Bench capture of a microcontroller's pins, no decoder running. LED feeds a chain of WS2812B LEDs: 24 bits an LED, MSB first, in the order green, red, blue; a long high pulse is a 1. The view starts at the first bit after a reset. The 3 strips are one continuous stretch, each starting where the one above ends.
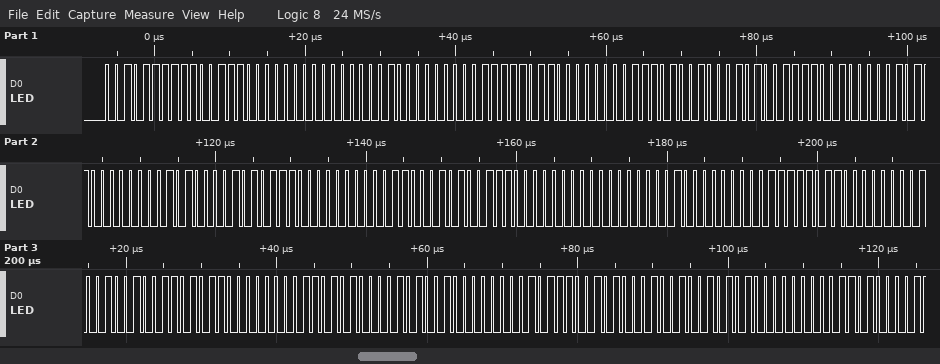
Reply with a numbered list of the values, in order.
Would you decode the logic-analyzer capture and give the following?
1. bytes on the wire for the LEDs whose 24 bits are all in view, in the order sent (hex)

1. 2F CE 00 02 00 FB 00 E9 14 F2 0B 00 A1 5C 00 C5 38 00 02 00 FB 00 92 6B 00 D4 29 00 B9 44 95 00 68
